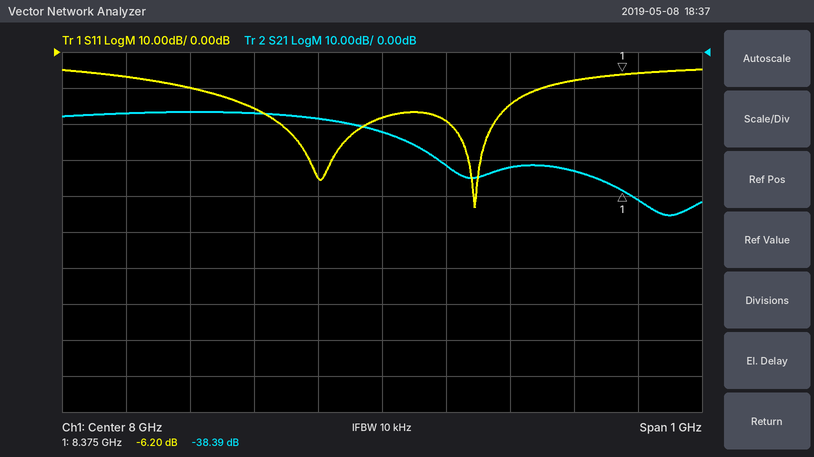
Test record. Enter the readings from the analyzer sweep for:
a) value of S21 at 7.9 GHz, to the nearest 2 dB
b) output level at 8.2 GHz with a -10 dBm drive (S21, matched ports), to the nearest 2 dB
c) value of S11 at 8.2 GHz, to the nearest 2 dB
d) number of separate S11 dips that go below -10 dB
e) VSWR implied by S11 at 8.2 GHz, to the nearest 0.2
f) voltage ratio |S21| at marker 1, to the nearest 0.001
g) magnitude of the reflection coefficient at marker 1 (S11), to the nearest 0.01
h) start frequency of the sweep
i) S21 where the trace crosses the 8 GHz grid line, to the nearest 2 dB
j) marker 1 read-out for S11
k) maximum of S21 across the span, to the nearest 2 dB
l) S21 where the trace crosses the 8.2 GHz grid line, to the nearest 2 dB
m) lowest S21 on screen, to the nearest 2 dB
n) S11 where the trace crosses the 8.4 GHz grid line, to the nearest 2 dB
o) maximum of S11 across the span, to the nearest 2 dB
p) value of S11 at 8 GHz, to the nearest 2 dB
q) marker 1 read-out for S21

-18 dB
-42 dBm
-14 dB
2
1.4
0.012
0.49
7.5 GHz
-22 dB
-6.20 dB
-16 dB
-32 dB
-46 dB
-6 dB
-4 dB
-18 dB
-38.39 dB
